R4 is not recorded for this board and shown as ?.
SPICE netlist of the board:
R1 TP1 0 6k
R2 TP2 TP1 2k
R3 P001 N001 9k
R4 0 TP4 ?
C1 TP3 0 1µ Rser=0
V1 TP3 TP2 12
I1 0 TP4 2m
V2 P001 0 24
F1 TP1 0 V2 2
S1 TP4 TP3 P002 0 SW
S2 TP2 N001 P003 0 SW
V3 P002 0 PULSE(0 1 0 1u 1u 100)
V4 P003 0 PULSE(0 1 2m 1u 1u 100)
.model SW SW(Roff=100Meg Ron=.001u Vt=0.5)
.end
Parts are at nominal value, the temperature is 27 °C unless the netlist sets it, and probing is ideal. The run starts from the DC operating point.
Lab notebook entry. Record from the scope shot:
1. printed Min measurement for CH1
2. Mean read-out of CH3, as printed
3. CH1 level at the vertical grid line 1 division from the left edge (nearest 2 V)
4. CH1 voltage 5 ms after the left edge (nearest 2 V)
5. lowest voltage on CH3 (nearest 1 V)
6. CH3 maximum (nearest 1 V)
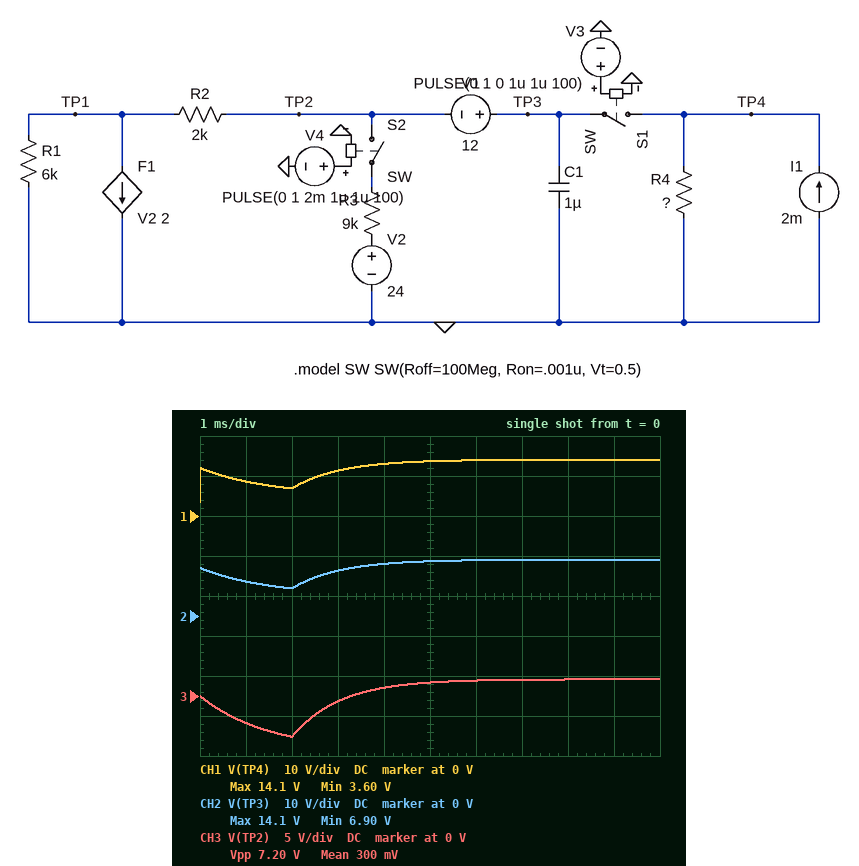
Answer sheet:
3.60 V
300 mV
8 V
14 V
-5 V
2 V
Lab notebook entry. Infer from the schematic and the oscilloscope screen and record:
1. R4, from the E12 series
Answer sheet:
1.8 kΩ
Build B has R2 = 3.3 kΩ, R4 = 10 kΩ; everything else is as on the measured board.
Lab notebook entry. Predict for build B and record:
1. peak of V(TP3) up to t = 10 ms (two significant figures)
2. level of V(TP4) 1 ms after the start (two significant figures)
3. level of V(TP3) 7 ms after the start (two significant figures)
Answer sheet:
27 V
13 V
26 V
